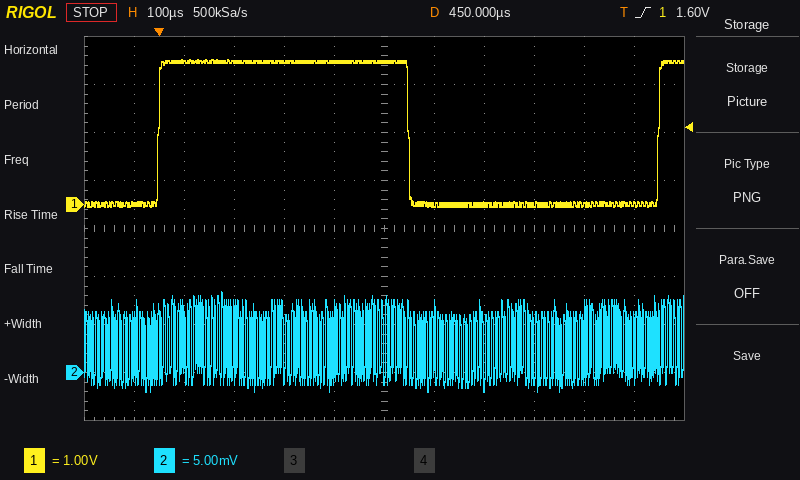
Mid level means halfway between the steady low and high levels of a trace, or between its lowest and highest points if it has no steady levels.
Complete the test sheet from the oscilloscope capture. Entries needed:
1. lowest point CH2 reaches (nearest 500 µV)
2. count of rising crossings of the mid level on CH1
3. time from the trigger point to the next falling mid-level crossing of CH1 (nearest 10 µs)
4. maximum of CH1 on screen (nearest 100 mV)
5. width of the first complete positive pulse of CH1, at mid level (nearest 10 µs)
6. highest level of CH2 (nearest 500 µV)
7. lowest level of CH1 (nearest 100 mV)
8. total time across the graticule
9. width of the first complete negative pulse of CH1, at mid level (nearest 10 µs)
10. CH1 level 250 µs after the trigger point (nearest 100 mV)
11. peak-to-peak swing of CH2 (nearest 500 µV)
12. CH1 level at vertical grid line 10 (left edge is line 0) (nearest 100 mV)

-2.0 mV
2
500 µs
3.0 V
500 µs
8.5 mV
0.0 V
1.2 ms
500 µs
3.0 V
10.5 mV
0.0 V
